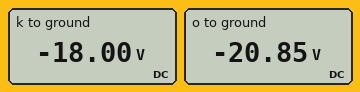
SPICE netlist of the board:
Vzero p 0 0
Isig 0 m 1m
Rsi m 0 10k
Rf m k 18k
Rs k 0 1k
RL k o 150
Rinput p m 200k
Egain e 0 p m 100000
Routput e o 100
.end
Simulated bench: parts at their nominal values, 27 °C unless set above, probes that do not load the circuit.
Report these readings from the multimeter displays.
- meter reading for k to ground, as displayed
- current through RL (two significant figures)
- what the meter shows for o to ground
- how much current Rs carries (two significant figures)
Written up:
-18.00 V
19 mA
-20.85 V
18 mA
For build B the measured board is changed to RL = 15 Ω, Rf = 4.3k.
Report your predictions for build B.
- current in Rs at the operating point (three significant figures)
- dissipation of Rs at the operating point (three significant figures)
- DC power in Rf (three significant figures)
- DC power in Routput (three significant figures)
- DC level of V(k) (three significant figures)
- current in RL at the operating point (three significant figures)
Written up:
4.30 mA
18.5 mW
4.30 mW
2.81 mW
-4.30 V
5.30 mA
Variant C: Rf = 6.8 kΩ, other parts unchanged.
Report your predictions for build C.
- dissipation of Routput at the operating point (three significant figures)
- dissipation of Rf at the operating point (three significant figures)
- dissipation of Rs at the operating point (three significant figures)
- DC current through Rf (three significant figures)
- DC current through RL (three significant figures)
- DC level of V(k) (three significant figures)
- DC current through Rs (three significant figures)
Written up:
6.08 mW
6.80 mW
46.2 mW
1.00 mA
7.80 mA
-6.80 V
6.80 mA
